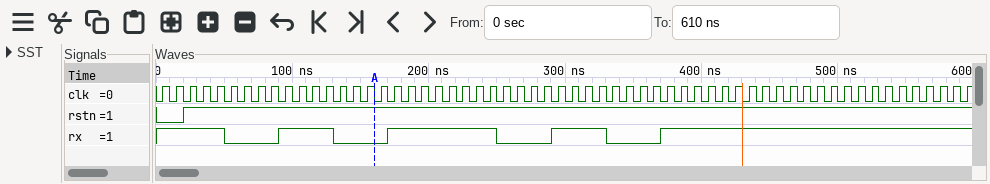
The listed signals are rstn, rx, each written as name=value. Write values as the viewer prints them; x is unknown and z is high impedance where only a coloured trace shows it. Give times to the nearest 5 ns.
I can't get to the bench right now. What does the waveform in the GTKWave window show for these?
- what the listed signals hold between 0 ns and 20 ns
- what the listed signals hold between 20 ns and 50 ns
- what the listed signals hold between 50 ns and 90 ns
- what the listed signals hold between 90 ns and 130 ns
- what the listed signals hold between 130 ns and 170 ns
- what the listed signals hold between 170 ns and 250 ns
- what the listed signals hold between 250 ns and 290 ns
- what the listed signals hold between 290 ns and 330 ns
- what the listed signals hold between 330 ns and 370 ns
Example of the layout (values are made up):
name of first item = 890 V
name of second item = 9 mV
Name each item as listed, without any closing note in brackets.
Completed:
what the listed signals hold between 0 ns and 20 ns = rstn=0, rx=1
what the listed signals hold between 20 ns and 50 ns = rstn=1, rx=1
what the listed signals hold between 50 ns and 90 ns = rstn=1, rx=0
what the listed signals hold between 90 ns and 130 ns = rstn=1, rx=1
what the listed signals hold between 130 ns and 170 ns = rstn=1, rx=0
what the listed signals hold between 170 ns and 250 ns = rstn=1, rx=1
what the listed signals hold between 250 ns and 290 ns = rstn=1, rx=0
what the listed signals hold between 290 ns and 330 ns = rstn=1, rx=1
what the listed signals hold between 330 ns and 370 ns = rstn=1, rx=0
